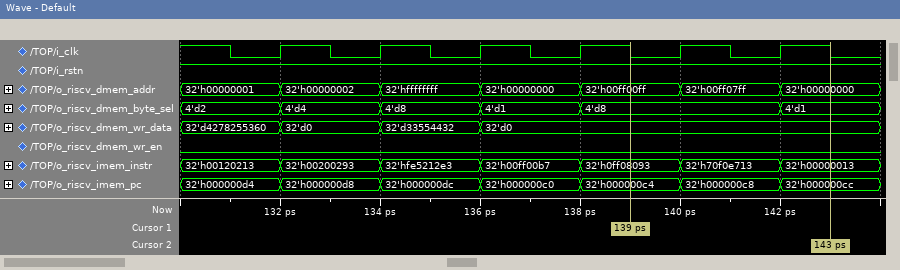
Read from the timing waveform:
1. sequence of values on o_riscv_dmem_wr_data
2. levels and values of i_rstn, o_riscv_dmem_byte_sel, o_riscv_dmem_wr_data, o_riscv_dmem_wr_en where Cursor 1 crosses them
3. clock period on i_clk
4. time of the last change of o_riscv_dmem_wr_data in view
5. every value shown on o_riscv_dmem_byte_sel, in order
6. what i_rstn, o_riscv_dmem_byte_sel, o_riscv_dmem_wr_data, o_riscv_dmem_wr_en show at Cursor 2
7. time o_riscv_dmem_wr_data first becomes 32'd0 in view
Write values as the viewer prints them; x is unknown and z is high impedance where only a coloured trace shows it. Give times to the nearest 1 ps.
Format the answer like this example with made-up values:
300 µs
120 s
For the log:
32'd4278255360, 32'd0, 32'd33554432, 32'd0
i_rstn=1, o_riscv_dmem_byte_sel=4'd8, o_riscv_dmem_wr_data=32'd0, o_riscv_dmem_wr_en=0
2 ps
136 ps
4'd2, 4'd4, 4'd8, 4'd1, 4'd8, 4'd1
i_rstn=1, o_riscv_dmem_byte_sel=4'd1, o_riscv_dmem_wr_data=32'd0, o_riscv_dmem_wr_en=0
132 ps
